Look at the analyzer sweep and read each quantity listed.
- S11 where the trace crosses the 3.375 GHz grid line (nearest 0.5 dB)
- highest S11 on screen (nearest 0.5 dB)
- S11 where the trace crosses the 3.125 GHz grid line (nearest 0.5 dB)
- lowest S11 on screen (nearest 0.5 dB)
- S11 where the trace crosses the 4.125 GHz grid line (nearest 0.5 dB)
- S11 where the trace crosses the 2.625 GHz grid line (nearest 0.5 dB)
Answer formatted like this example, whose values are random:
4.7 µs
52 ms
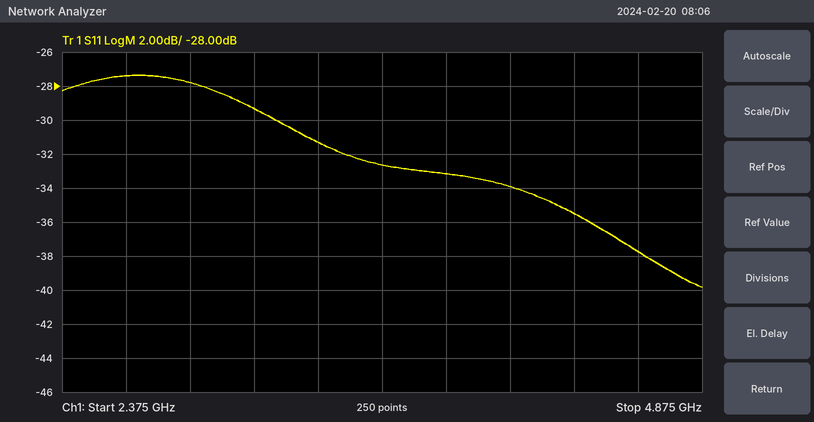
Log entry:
-31.5 dB
-27.5 dB
-29.5 dB
-40.0 dB
-34.0 dB
-27.5 dB
